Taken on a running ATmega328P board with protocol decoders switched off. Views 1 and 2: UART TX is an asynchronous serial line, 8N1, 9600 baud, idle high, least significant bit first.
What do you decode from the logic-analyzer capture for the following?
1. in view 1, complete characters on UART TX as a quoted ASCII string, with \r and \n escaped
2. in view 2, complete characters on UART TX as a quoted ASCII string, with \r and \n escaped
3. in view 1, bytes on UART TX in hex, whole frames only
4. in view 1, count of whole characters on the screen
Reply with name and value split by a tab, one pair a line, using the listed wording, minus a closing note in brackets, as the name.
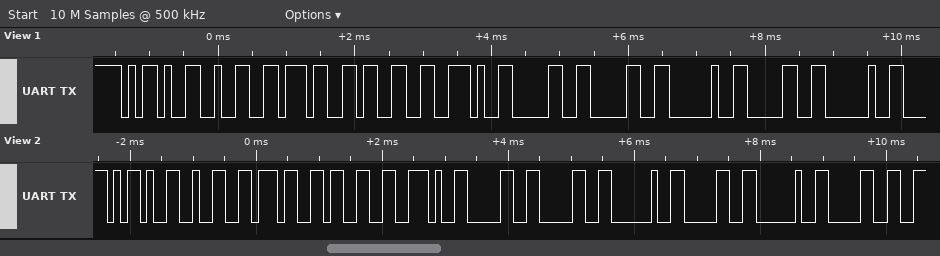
in view 1, complete characters on UART TX as a quoted ASCII string, with \r and \n escaped	"-273.00 0 "
in view 2, complete characters on UART TX as a quoted ASCII string, with \r and \n escaped	"-273.00 0 0"
in view 1, bytes on UART TX in hex, whole frames only	0x2D 0x32 0x37 0x33 0x2E 0x30 0x30 0x20 0x30 0x20
in view 1, count of whole characters on the screen	10
